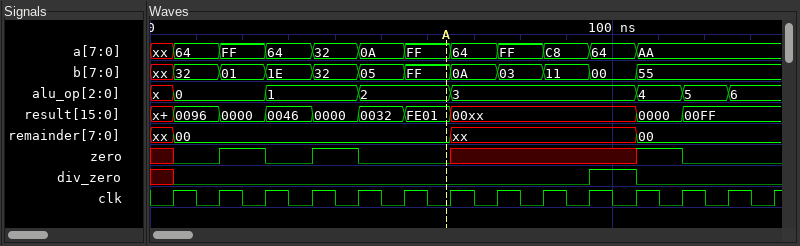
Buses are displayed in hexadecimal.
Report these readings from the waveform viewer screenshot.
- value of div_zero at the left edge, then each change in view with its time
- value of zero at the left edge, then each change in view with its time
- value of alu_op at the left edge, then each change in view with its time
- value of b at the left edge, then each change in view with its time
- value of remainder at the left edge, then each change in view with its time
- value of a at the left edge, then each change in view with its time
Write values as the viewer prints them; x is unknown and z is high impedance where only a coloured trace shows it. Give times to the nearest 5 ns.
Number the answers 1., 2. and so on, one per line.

1. x, 0 at 5 ns, 1 at 95 ns, 0 at 105 ns
2. x, 0 at 5 ns, 1 at 15 ns, 0 at 25 ns, 1 at 35 ns, 0 at 45 ns, x at 65 ns, 1 at 105 ns, 0 at 115 ns
3. x, 0 at 5 ns, 1 at 25 ns, 2 at 45 ns, 3 at 65 ns, 4 at 105 ns, 5 at 115 ns, 6 at 125 ns
4. xx, 32 at 5 ns, 01 at 15 ns, 1E at 25 ns, 32 at 35 ns, 05 at 45 ns, FF at 55 ns, 0A at 65 ns, 03 at 75 ns, 11 at 85 ns, 00 at 95 ns, 55 at 105 ns
5. xx, 00 at 5 ns, xx at 65 ns, 00 at 105 ns
6. xx, 64 at 5 ns, FF at 15 ns, 64 at 25 ns, 32 at 35 ns, 0A at 45 ns, FF at 55 ns, 64 at 65 ns, FF at 75 ns, C8 at 85 ns, 64 at 95 ns, AA at 105 ns
